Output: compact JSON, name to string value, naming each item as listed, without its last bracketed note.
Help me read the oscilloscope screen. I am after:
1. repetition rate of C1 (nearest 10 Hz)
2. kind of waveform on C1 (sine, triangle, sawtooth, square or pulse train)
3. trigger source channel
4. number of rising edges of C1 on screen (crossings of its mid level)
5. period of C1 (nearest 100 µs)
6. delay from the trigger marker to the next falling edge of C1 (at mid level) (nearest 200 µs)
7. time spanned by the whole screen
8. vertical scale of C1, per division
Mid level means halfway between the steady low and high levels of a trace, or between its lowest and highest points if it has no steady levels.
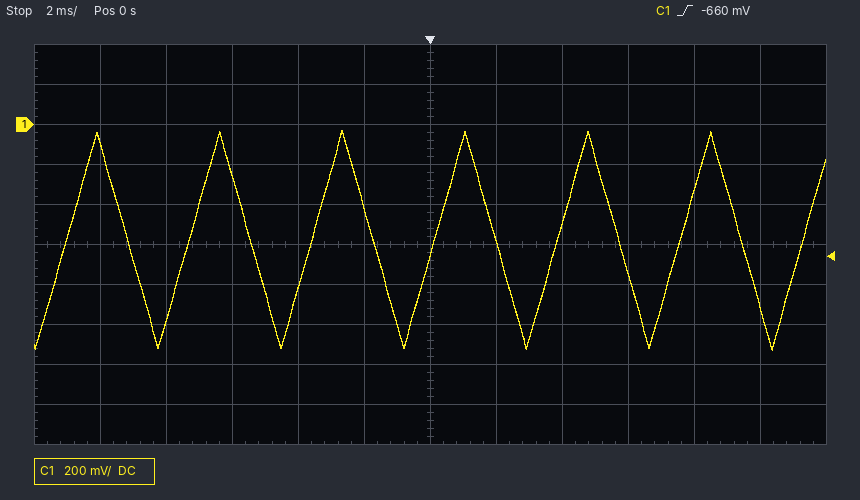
{"repetition rate of C1": "270 Hz", "kind of waveform on C1": "triangle", "trigger source channel": "C1", "number of rising edges of C1 on screen": "7", "period of C1": "3.7 ms", "delay from the trigger marker to the next falling edge of C1 (at mid level)": "2.0 ms", "time spanned by the whole screen": "24 ms", "vertical scale of C1, per division": "200 mV"}
